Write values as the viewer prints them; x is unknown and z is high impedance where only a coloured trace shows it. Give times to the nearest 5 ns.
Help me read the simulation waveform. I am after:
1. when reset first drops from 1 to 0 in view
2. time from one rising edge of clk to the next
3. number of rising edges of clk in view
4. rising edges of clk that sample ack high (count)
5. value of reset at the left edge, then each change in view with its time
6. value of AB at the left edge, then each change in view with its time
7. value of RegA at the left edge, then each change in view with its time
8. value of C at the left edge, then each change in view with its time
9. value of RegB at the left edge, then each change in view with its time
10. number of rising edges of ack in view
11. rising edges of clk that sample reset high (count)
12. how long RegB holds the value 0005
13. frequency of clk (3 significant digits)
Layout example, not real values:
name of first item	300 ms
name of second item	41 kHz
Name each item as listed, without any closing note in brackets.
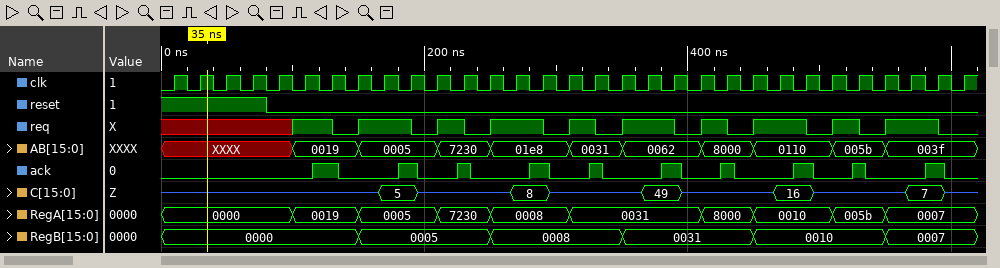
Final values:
when reset first drops from 1 to 0 in view	80 ns
time from one rising edge of clk to the next	20 ns
number of rising edges of clk in view	31
rising edges of clk that sample ack high	10
value of reset at the left edge, then each change in view with its time	1, 0 at 80 ns
value of AB at the left edge, then each change in view with its time	XXXX, 0019 at 100 ns, 0005 at 150 ns, 7230 at 210 ns, 01e8 at 250 ns, 0031 at 310 ns, 0062 at 350 ns, 8000 at 410 ns, 0110 at 450 ns, 005b at 510 ns, 003f at 550 ns
value of RegA at the left edge, then each change in view with its time	0000, 0019 at 100 ns, 0005 at 150 ns, 7230 at 210 ns, 0008 at 250 ns, 0031 at 310 ns, 8000 at 410 ns, 0010 at 450 ns, 005b at 510 ns, 0007 at 550 ns
value of C at the left edge, then each change in view with its time	z, 5 at 165 ns, z at 195 ns, 8 at 265 ns, z at 295 ns, 49 at 365 ns, z at 395 ns, 16 at 465 ns, z at 495 ns, 7 at 565 ns, z at 595 ns
value of RegB at the left edge, then each change in view with its time	0000, 0005 at 150 ns, 0008 at 250 ns, 0031 at 350 ns, 0010 at 450 ns, 0007 at 550 ns
number of rising edges of ack in view	10
rising edges of clk that sample reset high	4
how long RegB holds the value 0005	100 ns
frequency of clk	50.0 MHz
